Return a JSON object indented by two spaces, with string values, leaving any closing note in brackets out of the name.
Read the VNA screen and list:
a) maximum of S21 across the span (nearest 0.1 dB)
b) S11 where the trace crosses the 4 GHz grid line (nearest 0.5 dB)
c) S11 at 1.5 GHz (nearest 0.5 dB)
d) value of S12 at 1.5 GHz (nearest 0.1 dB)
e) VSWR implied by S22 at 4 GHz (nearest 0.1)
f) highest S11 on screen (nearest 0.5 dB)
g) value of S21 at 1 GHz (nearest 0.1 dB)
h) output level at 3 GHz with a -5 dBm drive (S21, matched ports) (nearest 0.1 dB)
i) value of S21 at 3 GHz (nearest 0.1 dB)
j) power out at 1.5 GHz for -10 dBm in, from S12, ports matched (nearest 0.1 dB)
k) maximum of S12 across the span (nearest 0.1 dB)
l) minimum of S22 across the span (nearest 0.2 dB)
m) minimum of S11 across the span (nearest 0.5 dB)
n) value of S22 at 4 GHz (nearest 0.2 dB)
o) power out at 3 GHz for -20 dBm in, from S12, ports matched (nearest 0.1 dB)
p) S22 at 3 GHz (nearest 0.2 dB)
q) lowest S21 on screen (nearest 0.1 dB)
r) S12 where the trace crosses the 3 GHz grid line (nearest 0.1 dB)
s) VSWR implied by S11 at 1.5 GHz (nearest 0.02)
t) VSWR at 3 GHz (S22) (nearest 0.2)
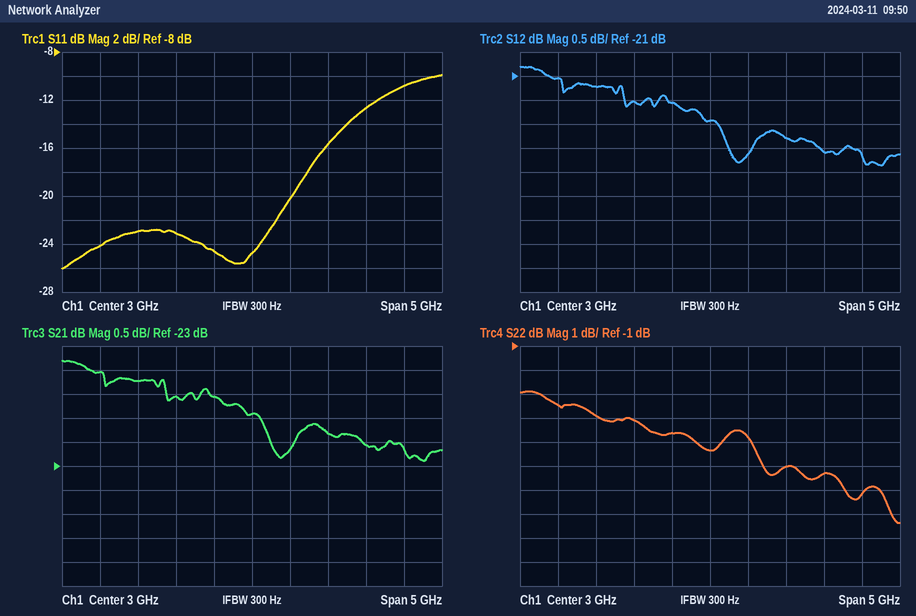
{
  "maximum of S21 across the span": "-20.8 dB",
  "S11 where the trace crosses the 4 GHz grid line": "-15.5 dB",
  "S11 at 1.5 GHz": "-23.0 dB",
  "value of S12 at 1.5 GHz": "-21.2 dB",
  "VSWR implied by S22 at 4 GHz": "3.0",
  "highest S11 on screen": "-10.0 dB",
  "value of S21 at 1 GHz": "-21.0 dB",
  "output level at 3 GHz with a -5 dBm drive (S21, matched ports)": "-26.9 dBm",
  "value of S21 at 3 GHz": "-21.9 dB",
  "power out at 1.5 GHz for -10 dBm in, from S12, ports matched": "-31.2 dBm",
  "maximum of S12 across the span": "-20.8 dB",
  "minimum of S22 across the span": "-8.4 dB",
  "minimum of S11 across the span": "-26.0 dB",
  "value of S22 at 4 GHz": "-6.0 dB",
  "power out at 3 GHz for -20 dBm in, from S12, ports matched": "-41.9 dBm",
  "S22 at 3 GHz": "-5.4 dB",
  "lowest S21 on screen": "-22.9 dB",
  "S12 where the trace crosses the 3 GHz grid line": "-21.9 dB",
  "VSWR implied by S11 at 1.5 GHz": "1.16",
  "VSWR at 3 GHz (S22)": "3.4"
}
